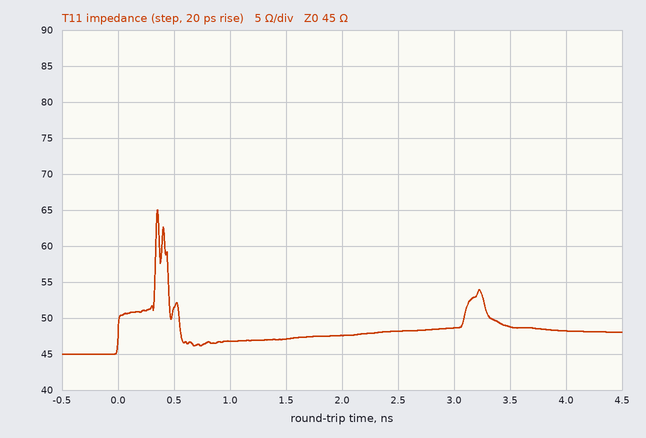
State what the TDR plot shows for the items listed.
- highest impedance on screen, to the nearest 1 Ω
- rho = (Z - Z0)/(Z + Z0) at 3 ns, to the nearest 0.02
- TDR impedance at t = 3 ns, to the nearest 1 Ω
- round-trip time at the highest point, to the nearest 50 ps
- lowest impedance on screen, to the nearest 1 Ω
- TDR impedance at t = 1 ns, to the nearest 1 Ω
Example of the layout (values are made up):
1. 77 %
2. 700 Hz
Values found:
1. 65 Ω
2. +0.04
3. 49 Ω
4. 350 ps
5. 45 Ω
6. 47 Ω
